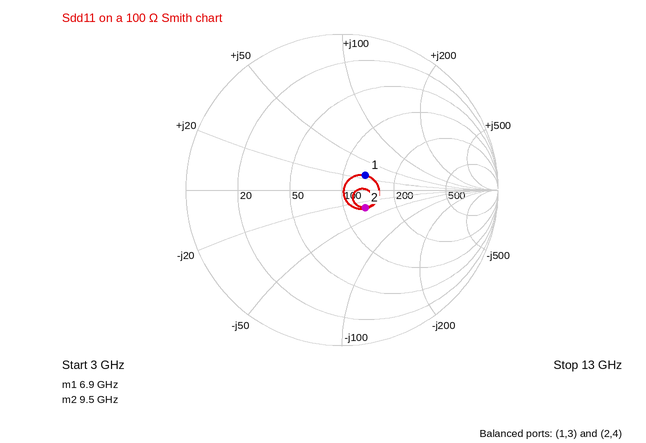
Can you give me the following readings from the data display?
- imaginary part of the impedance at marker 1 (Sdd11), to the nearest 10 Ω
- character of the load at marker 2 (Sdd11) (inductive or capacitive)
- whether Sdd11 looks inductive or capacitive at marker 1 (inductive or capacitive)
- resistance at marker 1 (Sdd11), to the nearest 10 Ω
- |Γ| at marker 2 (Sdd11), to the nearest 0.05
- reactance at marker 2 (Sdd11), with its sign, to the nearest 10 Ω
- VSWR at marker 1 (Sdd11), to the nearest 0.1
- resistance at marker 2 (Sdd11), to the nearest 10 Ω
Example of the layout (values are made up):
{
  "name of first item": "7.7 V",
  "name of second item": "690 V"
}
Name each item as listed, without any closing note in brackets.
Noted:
{
  "imaginary part of the impedance at marker 1 (Sdd11), to the nearest 10 Ω": "+30 Ω",
  "character of the load at marker 2 (Sdd11)": "capacitive",
  "whether Sdd11 looks inductive or capacitive at marker 1": "inductive",
  "resistance at marker 1 (Sdd11), to the nearest 10 Ω": "130 Ω",
  "|Γ| at marker 2 (Sdd11), to the nearest 0.05": "0.20",
  "reactance at marker 2 (Sdd11), with its sign, to the nearest 10 Ω": "-30 Ω",
  "VSWR at marker 1 (Sdd11), to the nearest 0.1": "1.4",
  "resistance at marker 2 (Sdd11), to the nearest 10 Ω": "130 Ω"
}
